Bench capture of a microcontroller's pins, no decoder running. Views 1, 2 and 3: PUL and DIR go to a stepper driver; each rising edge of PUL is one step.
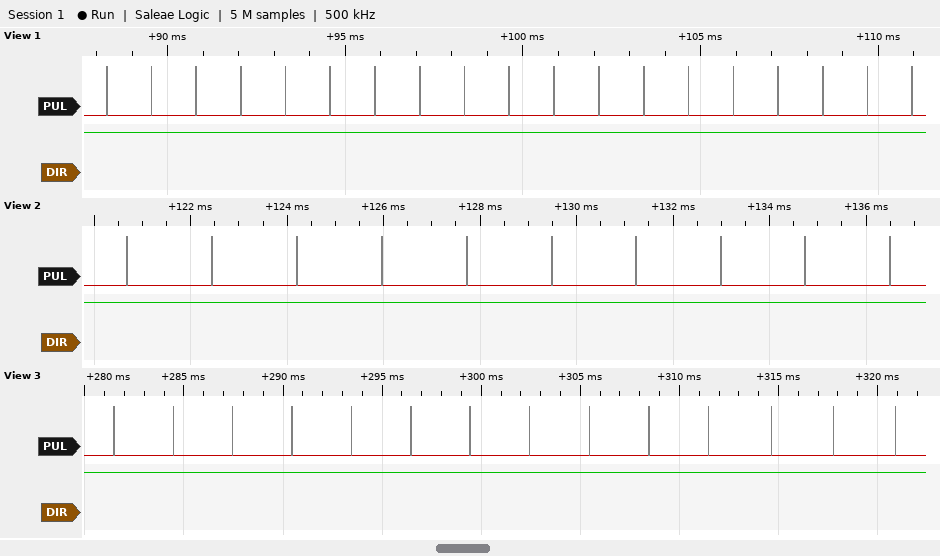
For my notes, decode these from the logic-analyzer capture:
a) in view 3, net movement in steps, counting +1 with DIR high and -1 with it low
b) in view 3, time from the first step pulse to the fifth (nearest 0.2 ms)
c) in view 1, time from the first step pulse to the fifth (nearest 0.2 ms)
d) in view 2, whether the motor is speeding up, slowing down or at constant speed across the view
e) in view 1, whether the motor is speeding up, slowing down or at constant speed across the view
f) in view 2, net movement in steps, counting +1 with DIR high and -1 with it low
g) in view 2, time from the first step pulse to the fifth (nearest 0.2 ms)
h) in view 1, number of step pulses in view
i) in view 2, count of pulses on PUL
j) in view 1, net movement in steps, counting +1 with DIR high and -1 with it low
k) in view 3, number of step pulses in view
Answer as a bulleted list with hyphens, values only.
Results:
- +14
- 12.0 ms
- 5.0 ms
- constant speed
- constant speed
- +10
- 7.0 ms
- 19
- 10
- +19
- 14
